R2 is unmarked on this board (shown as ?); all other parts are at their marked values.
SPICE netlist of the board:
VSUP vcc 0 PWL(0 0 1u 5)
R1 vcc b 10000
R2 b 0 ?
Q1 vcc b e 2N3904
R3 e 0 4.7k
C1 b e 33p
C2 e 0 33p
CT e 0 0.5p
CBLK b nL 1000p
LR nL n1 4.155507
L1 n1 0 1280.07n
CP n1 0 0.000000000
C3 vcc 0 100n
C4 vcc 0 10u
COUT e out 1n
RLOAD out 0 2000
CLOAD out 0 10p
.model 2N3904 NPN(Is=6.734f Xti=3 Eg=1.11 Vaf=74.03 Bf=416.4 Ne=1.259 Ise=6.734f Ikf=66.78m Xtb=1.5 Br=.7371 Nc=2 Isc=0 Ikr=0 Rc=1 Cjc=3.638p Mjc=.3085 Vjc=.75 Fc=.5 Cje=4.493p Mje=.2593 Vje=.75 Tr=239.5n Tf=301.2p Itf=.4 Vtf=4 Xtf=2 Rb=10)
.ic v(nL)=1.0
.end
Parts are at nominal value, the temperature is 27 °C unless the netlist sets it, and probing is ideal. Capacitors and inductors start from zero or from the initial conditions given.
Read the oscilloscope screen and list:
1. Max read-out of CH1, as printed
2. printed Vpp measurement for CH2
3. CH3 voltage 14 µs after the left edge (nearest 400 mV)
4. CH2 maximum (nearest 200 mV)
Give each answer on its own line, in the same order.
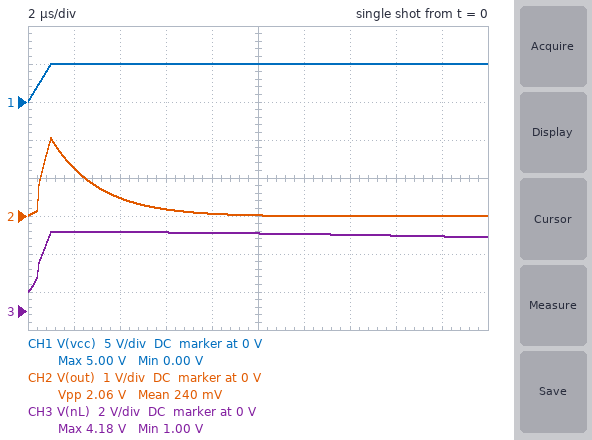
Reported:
5.00 V
2.06 V
4.0 V
2.0 V
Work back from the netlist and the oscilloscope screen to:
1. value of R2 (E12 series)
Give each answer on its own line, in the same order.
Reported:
18 kΩ
